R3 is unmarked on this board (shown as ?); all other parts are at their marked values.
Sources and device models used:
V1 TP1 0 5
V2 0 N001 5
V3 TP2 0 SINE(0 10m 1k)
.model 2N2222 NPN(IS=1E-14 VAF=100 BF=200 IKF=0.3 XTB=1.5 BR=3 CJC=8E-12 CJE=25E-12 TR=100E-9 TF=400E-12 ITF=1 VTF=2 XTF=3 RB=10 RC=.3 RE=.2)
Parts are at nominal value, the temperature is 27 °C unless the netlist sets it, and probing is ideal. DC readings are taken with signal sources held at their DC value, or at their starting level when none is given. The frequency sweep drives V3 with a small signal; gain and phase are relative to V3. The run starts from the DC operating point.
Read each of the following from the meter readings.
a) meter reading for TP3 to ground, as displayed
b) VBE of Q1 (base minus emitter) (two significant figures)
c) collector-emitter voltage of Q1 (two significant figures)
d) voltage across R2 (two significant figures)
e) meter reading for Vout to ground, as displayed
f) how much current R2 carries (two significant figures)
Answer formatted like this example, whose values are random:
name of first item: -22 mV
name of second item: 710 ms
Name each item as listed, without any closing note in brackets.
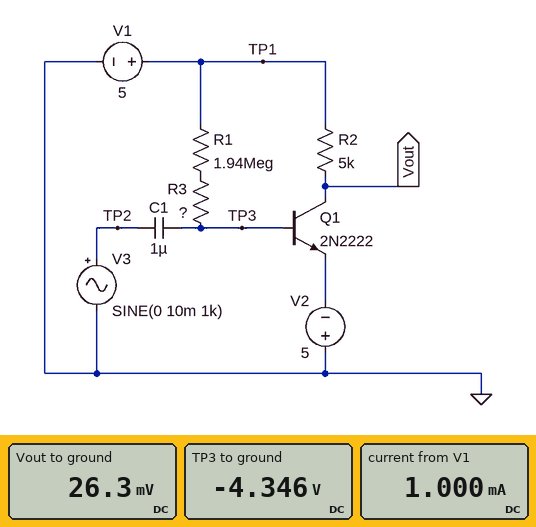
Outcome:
meter reading for TP3 to ground, as displayed: -4.346 V
VBE of Q1 (base minus emitter): 650 mV
collector-emitter voltage of Q1: 5.0 V
voltage across R2: 5.0 V
meter reading for Vout to ground, as displayed: 26.3 mV
how much current R2 carries: 990 µA
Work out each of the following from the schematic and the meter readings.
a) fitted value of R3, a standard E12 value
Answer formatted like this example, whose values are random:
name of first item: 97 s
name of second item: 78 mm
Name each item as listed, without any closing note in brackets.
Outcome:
fitted value of R3, a standard E12 value: 15 kΩ
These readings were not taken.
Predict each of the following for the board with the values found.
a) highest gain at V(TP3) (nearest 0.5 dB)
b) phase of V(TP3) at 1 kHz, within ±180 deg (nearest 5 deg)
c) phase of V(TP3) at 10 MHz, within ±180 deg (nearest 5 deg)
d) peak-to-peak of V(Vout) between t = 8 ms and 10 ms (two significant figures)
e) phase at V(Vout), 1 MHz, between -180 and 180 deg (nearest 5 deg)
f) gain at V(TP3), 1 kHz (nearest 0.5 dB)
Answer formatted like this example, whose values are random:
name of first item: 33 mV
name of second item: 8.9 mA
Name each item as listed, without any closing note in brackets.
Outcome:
highest gain at V(TP3): 0 dB
phase of V(TP3) at 1 kHz, within ±180 deg: 0 deg
phase of V(TP3) at 10 MHz, within ±180 deg: 0 deg
peak-to-peak of V(Vout) between t = 8 ms and 10 ms: 3.6 V
phase at V(Vout), 1 MHz, between -180 and 180 deg: 170 deg
gain at V(TP3), 1 kHz: 0 dB
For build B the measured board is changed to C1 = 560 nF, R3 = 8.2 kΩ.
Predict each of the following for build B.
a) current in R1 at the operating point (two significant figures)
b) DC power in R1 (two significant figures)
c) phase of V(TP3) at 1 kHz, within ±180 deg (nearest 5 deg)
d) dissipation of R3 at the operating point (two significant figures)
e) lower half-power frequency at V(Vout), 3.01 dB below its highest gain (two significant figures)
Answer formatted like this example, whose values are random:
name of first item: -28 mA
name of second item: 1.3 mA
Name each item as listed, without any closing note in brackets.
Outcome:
current in R1 at the operating point: 4.8 µA
DC power in R1: 45 µW
phase of V(TP3) at 1 kHz, within ±180 deg: 5 deg
dissipation of R3 at the operating point: 190 nW
lower half-power frequency at V(Vout), 3.01 dB below its highest gain: 52 Hz
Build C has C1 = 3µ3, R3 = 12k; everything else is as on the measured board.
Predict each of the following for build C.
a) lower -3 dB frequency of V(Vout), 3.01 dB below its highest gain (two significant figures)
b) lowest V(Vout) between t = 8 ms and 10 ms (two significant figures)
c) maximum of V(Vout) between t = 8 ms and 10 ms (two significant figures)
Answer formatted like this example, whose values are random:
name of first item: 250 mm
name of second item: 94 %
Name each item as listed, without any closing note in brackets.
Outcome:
lower -3 dB frequency of V(Vout), 3.01 dB below its highest gain: 8.9 Hz
lowest V(Vout) between t = 8 ms and 10 ms: -2.0 V
maximum of V(Vout) between t = 8 ms and 10 ms: 1.6 V
